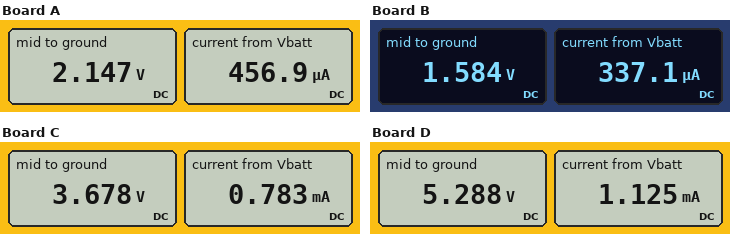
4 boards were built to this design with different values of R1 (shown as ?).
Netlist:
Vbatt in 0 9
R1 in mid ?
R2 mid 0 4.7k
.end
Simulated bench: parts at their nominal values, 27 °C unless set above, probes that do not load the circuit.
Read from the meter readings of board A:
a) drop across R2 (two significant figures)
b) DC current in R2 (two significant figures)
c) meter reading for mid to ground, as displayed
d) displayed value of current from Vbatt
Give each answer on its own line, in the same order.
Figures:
2.1 V
460 µA
2.147 V
456.9 µA
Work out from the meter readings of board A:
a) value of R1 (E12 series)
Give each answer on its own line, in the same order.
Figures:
15 kΩ
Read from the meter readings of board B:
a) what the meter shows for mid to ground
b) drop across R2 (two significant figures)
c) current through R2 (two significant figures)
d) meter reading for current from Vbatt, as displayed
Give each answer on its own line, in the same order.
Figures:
1.584 V
1.6 V
340 µA
337.1 µA
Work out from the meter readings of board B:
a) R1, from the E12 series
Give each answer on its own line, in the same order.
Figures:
22 kΩ
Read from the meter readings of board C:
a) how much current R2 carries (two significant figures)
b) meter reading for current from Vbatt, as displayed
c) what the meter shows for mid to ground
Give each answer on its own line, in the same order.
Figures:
780 µA
0.783 mA
3.678 V
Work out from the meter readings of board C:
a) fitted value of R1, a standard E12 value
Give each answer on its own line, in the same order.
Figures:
6.8 kΩ
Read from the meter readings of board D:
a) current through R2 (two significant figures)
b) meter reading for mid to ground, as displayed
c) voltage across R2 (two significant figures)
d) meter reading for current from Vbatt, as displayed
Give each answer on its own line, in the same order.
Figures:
1.1 mA
5.288 V
5.3 V
1.125 mA
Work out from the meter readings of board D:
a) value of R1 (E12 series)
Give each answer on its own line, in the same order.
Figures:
3.3 kΩ
